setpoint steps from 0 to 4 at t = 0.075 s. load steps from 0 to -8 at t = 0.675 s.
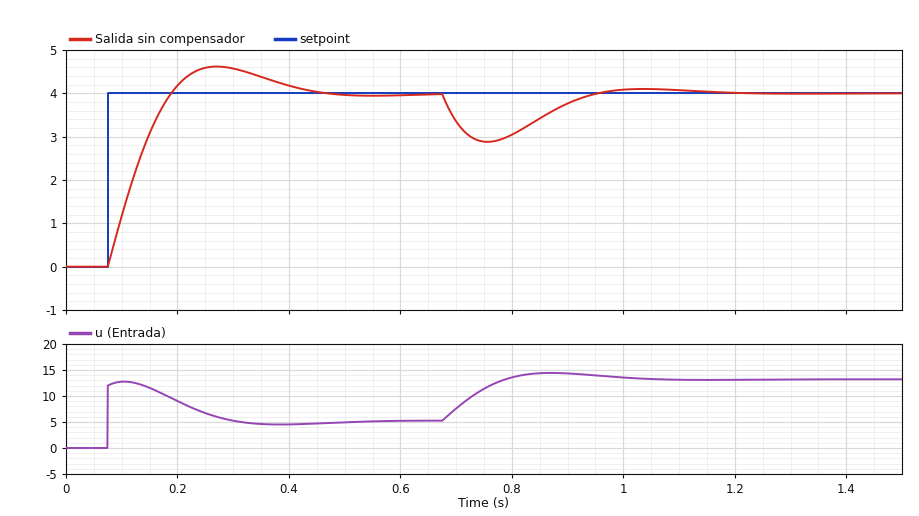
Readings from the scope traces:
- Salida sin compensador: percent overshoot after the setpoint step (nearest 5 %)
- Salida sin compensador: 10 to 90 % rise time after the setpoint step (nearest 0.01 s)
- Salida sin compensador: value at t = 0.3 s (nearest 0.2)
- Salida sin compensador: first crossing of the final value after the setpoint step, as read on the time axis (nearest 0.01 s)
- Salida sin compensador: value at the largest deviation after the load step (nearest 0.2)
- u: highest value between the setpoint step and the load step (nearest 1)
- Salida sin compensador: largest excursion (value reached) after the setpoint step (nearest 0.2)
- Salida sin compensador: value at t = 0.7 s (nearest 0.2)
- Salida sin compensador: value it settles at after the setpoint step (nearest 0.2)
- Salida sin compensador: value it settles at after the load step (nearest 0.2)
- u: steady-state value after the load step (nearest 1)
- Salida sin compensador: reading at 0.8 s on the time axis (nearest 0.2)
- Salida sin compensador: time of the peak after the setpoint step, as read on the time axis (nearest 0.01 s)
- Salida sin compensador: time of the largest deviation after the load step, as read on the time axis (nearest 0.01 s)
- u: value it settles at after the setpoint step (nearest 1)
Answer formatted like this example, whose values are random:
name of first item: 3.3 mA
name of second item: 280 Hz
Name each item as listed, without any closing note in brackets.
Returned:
Salida sin compensador: percent overshoot after the setpoint step: 15 %
Salida sin compensador: 10 to 90 % rise time after the setpoint step: 0.09 s
Salida sin compensador: value at t = 0.3 s: 4.6
Salida sin compensador: first crossing of the final value after the setpoint step, as read on the time axis: 0.19 s
Salida sin compensador: value at the largest deviation after the load step: 2.8
u: highest value between the setpoint step and the load step: 13
Salida sin compensador: largest excursion (value reached) after the setpoint step: 4.6
Salida sin compensador: value at t = 0.7 s: 3.4
Salida sin compensador: value it settles at after the setpoint step: 4.0
Salida sin compensador: value it settles at after the load step: 4.0
u: steady-state value after the load step: 13
Salida sin compensador: reading at 0.8 s on the time axis: 3.0
Salida sin compensador: time of the peak after the setpoint step, as read on the time axis: 0.27 s
Salida sin compensador: time of the largest deviation after the load step, as read on the time axis: 0.76 s
u: value it settles at after the setpoint step: 5
